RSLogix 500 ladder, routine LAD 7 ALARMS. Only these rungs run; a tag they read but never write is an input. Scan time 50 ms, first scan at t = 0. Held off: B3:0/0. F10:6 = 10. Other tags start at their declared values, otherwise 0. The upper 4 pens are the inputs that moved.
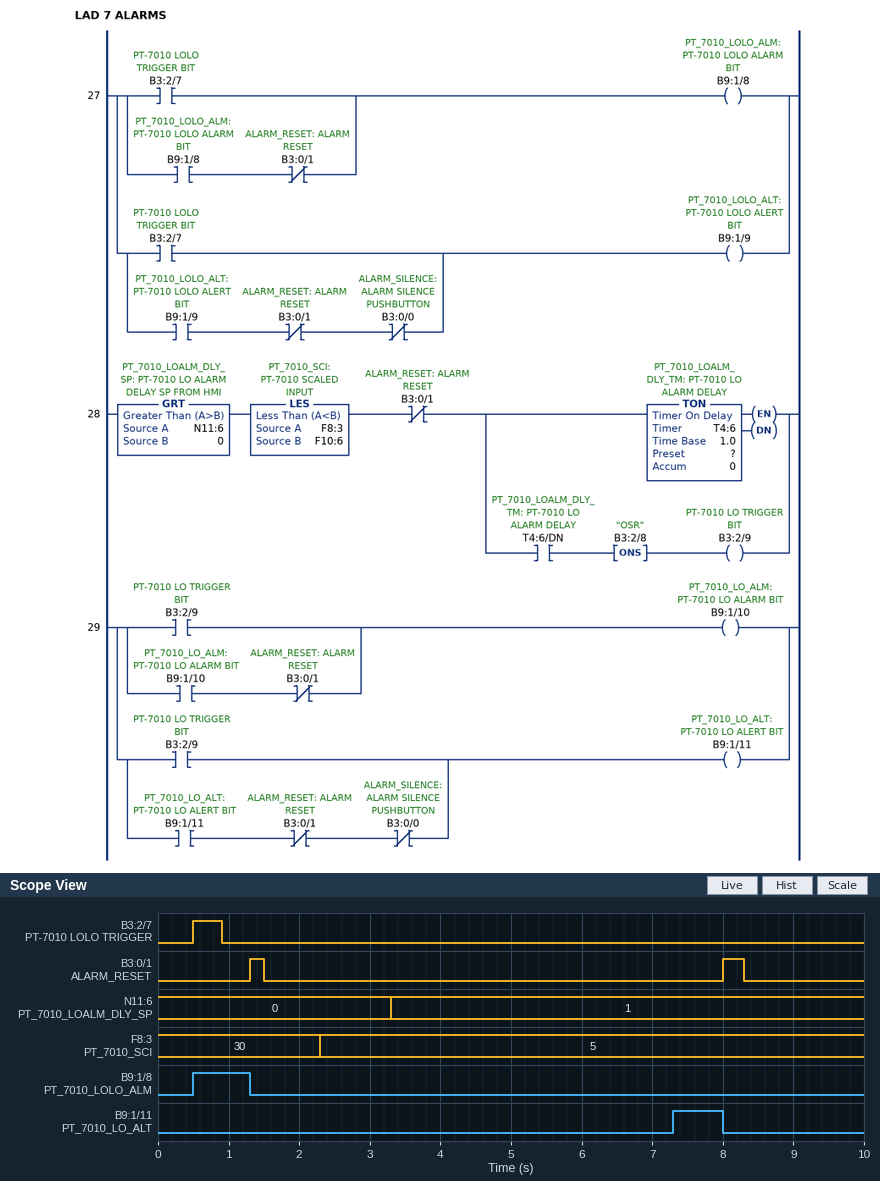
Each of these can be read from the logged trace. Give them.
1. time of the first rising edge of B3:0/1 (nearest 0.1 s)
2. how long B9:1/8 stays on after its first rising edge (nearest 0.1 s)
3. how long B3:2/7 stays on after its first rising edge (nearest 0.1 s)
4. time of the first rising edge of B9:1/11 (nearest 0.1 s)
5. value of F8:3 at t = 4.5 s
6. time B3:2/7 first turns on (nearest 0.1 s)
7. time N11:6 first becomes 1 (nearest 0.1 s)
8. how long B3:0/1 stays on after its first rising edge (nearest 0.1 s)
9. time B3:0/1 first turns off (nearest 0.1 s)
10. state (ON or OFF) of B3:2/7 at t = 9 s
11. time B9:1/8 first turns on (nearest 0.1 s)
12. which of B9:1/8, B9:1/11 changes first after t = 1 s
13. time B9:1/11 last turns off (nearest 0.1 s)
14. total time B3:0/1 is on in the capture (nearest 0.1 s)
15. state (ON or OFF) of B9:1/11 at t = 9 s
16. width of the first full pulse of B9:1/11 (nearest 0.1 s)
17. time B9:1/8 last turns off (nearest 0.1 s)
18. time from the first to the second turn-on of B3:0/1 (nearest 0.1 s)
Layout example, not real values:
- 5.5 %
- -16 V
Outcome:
- 1.3 s
- 0.8 s
- 0.4 s
- 7.3 s
- 5
- 0.5 s
- 3.3 s
- 0.2 s
- 1.5 s
- OFF
- 0.5 s
- B9:1/8
- 8.0 s
- 0.5 s
- OFF
- 0.7 s
- 1.3 s
- 6.7 s
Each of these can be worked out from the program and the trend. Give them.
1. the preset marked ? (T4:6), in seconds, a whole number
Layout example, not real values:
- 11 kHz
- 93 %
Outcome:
- 4 s
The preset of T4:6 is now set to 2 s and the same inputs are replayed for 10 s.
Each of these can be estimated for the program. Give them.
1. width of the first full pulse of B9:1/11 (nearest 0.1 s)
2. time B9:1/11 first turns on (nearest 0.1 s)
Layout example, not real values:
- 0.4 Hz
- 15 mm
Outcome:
- 2.7 s
- 5.3 s
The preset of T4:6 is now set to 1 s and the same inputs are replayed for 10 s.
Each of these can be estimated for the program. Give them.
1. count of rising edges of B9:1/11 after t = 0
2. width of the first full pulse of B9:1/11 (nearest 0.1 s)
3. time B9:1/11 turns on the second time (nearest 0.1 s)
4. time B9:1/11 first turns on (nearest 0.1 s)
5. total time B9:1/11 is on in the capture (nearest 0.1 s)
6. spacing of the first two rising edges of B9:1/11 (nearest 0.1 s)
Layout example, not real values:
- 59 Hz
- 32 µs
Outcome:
- 2
- 3.7 s
- 9.3 s
- 4.3 s
- 4.4 s
- 5.0 s
